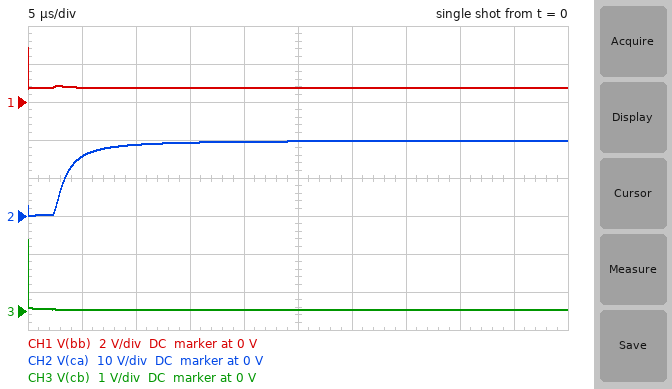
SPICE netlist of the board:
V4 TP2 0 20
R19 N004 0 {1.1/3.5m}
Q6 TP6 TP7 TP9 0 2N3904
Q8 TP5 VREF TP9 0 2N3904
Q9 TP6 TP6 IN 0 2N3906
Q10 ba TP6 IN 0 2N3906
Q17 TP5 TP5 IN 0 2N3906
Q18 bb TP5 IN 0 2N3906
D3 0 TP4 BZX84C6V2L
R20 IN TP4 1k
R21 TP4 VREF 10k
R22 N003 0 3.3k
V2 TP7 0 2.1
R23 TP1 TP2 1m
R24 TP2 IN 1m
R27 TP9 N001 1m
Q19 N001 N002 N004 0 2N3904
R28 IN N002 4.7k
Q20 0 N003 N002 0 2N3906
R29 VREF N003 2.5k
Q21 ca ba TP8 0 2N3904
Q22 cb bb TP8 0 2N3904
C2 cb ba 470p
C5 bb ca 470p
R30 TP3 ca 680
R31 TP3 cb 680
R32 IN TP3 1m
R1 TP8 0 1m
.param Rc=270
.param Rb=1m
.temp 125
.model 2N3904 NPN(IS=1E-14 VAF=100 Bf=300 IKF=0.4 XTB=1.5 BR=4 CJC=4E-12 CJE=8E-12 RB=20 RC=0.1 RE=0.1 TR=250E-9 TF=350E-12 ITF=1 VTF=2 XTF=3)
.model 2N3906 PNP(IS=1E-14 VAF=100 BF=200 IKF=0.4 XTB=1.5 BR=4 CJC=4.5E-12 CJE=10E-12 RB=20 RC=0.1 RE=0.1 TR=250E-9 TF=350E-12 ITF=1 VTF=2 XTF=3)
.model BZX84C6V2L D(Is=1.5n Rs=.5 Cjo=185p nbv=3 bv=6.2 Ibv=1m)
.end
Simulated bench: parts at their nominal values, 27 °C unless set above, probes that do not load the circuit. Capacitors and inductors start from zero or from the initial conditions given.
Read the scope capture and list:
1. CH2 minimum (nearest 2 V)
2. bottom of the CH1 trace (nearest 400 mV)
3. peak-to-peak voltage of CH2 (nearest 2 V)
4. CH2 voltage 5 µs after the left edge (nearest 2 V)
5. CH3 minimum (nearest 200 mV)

0 V
800 mV
20 V
16 V
0 V
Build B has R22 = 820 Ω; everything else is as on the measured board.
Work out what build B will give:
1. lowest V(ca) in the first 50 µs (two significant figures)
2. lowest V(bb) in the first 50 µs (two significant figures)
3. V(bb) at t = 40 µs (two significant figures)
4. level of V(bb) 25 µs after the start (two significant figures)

39 mV
420 mV
430 mV
450 mV
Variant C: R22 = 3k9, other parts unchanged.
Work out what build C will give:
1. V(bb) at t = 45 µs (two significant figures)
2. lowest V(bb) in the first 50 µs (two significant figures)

750 mV
720 mV
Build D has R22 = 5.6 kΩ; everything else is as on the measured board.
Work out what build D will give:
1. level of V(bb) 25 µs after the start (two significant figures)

790 mV
